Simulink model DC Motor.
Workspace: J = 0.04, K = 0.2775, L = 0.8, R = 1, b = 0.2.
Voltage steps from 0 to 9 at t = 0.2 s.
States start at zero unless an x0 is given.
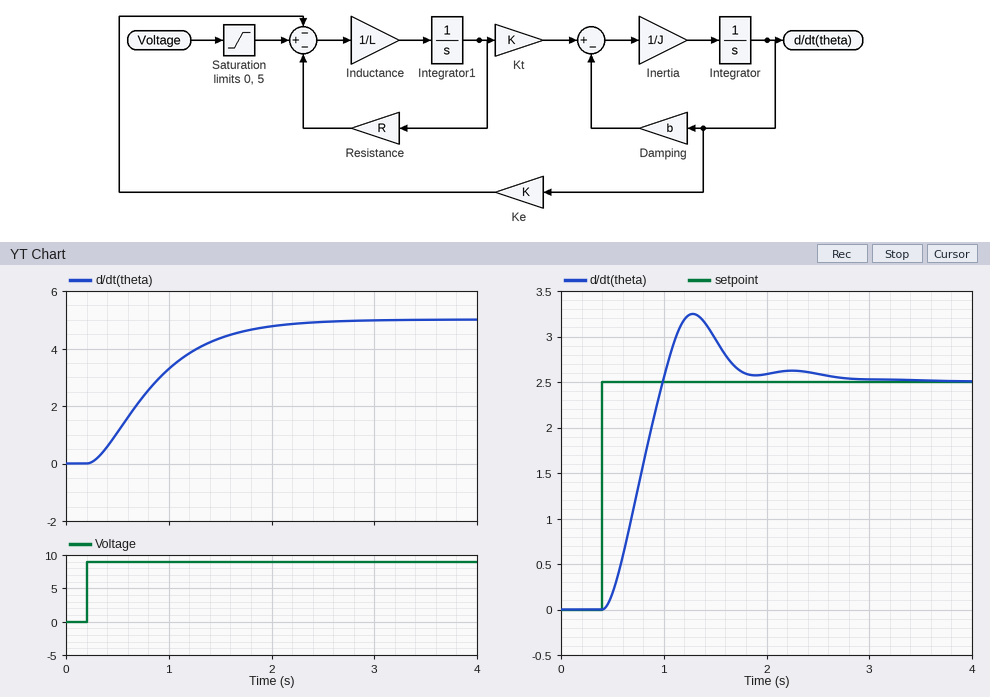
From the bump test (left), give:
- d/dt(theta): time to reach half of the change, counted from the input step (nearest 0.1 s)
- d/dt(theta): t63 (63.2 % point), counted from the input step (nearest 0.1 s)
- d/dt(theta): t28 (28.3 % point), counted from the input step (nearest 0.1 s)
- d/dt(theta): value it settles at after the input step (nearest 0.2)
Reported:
0.6 s
0.8 s
0.4 s
5.0
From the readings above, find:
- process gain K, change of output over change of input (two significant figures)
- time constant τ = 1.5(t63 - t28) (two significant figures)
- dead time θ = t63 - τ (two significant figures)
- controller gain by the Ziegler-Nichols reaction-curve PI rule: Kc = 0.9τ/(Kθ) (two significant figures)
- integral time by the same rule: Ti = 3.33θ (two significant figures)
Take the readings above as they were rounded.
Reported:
0.56
0.60 s
0.20 s
4.8
0.67 s
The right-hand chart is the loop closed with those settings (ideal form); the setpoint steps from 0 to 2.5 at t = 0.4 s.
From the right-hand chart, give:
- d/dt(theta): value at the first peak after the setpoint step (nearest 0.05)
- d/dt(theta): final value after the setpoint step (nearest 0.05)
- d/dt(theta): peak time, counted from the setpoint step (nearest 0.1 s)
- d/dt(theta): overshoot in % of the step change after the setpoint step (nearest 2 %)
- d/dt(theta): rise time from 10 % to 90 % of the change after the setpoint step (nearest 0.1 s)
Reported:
3.25
2.50
0.9 s
30 %
0.4 s
